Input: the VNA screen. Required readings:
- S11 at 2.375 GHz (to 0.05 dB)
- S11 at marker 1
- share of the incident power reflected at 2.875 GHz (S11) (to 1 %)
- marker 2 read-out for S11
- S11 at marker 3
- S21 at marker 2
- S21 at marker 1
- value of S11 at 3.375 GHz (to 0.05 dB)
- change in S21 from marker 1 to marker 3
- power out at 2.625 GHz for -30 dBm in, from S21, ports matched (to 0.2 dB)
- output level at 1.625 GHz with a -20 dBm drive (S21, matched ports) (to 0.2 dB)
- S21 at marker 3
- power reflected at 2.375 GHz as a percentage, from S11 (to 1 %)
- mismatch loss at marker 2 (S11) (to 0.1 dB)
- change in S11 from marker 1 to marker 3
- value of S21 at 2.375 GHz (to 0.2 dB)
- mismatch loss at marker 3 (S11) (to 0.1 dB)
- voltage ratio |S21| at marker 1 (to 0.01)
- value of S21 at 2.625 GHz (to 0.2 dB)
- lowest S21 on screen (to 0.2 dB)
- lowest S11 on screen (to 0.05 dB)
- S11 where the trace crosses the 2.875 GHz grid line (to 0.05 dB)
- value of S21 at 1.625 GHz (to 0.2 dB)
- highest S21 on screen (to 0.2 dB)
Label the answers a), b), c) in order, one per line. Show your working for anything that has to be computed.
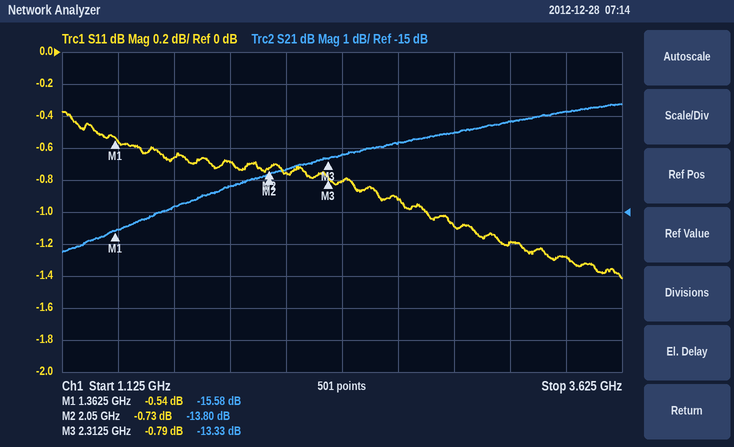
a) -0.80 dB
b) -0.54 dB
c) 10^(-1.1/10) ≈ 78 %
d) -0.73 dB
e) -0.79 dB
f) -13.80 dB
g) -15.58 dB
h) -1.30 dB
i) -13.33 − (-15.58) = 2.25 dB
j) -30 dBm + (-12.8 dB) = -42.8 dBm
k) -20 dBm + (-14.8 dB) = -34.8 dBm
l) -13.33 dB
m) 10^(-0.8/10) ≈ 83 %
n) −10 log10(1 − 10^(-0.73/10)) ≈ 8.1 dB
o) -0.79 − (-0.54) = -0.25 dB
p) -13.2 dB
q) −10 log10(1 − 10^(-0.79/10)) ≈ 7.8 dB
r) 10^(-15.58/20) ≈ 0.17
s) -12.8 dB
t) -16.2 dB
u) -1.40 dB
v) -1.10 dB
w) -14.8 dB
x) -11.6 dB
